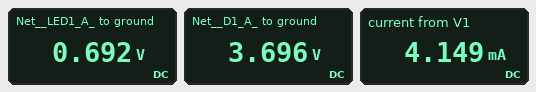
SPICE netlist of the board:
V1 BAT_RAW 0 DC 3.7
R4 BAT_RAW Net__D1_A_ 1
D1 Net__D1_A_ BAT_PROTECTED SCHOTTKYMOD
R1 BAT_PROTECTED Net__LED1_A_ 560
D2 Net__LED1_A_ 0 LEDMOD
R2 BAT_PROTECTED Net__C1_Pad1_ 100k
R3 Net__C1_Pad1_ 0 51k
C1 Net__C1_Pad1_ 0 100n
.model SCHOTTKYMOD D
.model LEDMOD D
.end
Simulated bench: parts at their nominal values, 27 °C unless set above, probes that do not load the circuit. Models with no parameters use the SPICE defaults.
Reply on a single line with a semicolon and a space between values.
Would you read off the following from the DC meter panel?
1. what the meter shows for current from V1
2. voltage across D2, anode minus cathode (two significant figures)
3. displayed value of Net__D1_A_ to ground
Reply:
4.149 mA; 690 mV; 3.696 V
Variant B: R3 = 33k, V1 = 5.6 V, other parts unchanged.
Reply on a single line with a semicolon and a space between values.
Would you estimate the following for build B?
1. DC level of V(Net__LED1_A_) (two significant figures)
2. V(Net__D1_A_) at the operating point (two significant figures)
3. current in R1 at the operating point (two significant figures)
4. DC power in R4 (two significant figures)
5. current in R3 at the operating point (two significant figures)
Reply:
710 mV; 5.6 V; 7.5 mA; 56 µW; 37 µA
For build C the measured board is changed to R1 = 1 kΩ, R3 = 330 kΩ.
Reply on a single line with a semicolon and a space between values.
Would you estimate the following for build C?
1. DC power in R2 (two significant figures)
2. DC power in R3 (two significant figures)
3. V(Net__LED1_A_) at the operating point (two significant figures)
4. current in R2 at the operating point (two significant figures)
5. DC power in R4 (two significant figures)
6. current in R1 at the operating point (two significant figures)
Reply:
4.9 µW; 16 µW; 680 mV; 7.0 µA; 5.5 µW; 2.3 mA
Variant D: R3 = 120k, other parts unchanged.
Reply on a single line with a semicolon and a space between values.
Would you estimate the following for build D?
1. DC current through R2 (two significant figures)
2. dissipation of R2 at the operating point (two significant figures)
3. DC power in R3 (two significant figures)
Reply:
14 µA; 19 µW; 22 µW
